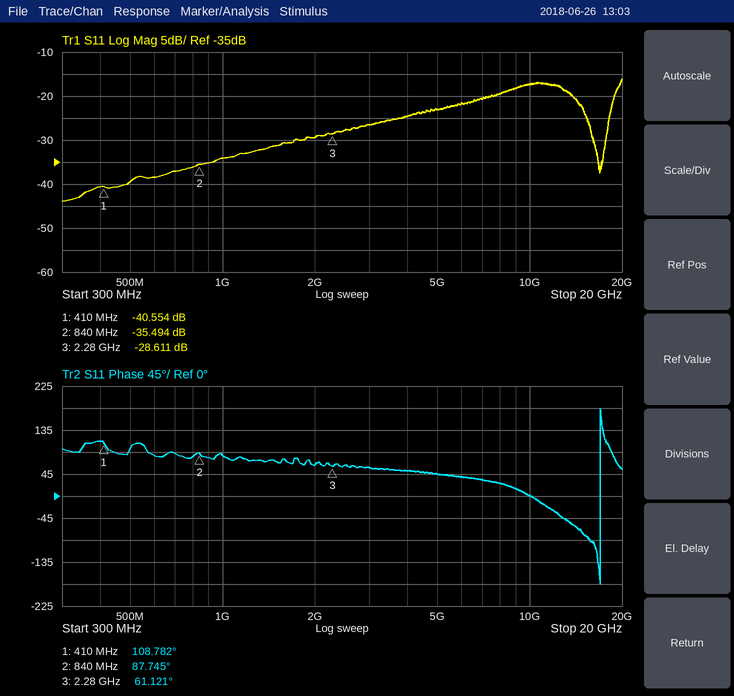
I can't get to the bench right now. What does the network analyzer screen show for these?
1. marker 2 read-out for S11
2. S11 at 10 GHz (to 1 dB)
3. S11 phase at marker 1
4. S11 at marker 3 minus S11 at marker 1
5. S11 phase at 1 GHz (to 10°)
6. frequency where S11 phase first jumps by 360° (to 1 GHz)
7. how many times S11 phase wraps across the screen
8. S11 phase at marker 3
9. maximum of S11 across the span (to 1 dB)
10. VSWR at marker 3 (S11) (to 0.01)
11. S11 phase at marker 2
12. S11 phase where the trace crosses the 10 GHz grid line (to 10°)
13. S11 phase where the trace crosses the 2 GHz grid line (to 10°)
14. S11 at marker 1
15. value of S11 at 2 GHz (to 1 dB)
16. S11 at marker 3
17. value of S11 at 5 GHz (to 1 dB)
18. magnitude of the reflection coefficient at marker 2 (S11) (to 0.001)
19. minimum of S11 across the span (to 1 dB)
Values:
-35.494 dB
-17 dB
108.782°
11.943 dB
80°
17 GHz
1
61.121°
-16 dB
1.08
87.745°
0°
60°
-40.554 dB
-29 dB
-28.611 dB
-23 dB
0.017
-44 dB
